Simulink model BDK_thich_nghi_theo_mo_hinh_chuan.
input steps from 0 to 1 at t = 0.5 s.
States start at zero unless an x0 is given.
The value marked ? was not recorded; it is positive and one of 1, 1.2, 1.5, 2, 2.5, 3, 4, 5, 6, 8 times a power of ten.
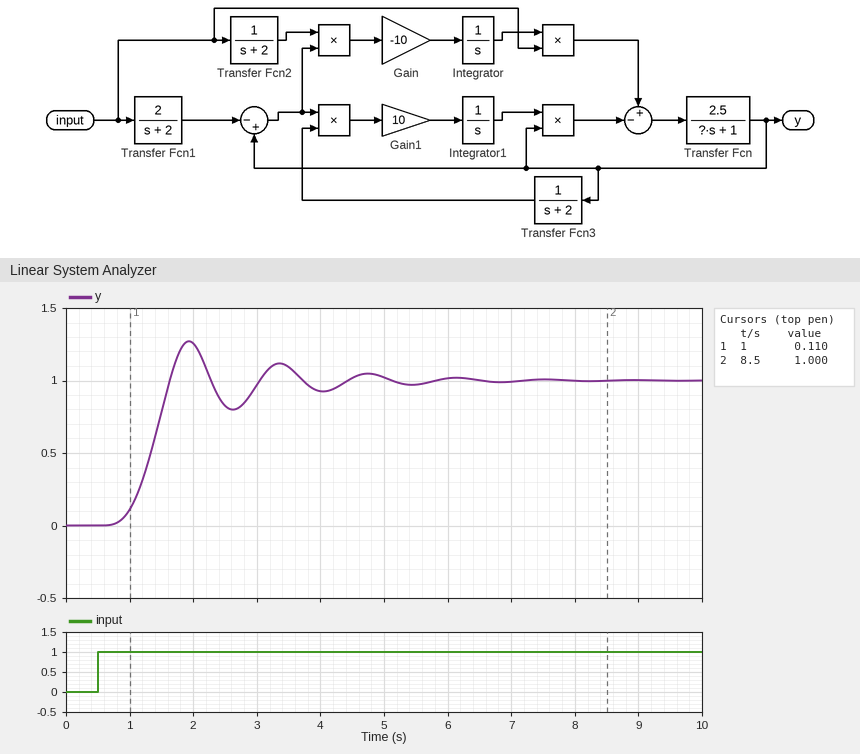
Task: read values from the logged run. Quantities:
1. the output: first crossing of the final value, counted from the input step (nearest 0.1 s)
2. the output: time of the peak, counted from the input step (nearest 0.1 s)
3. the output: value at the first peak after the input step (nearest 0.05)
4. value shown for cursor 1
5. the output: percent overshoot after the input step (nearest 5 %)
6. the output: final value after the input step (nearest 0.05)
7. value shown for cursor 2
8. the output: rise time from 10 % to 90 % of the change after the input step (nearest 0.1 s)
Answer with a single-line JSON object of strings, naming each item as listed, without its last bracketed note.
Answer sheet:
{"the output: first crossing of the final value, counted from the input step": "1.1 s", "the output: time of the peak, counted from the input step": "1.4 s", "the output: value at the first peak after the input step": "1.25", "value shown for cursor 1": "0.110", "the output: percent overshoot after the input step": "25 %", "the output: final value after the input step": "1.00", "value shown for cursor 2": "1.000", "the output: rise time from 10 % to 90 % of the change after the input step": "0.6 s"}
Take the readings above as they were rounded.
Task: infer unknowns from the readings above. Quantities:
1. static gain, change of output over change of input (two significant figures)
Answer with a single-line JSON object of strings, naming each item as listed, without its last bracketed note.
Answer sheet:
{"static gain, change of output over change of input": "1.0"}
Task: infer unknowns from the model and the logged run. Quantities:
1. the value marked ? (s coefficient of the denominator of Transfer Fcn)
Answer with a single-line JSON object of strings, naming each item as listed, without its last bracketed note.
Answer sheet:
{"the value marked ?": "1.2"}
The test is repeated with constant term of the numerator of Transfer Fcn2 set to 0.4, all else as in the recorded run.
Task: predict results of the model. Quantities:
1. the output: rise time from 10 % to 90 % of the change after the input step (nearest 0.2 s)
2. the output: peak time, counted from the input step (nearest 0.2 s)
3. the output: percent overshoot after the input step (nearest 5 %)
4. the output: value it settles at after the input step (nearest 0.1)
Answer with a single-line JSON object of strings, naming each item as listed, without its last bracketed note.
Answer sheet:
{"the output: rise time from 10 % to 90 % of the change after the input step": "0.8 s", "the output: peak time, counted from the input step": "1.8 s", "the output: percent overshoot after the input step": "30 %", "the output: value it settles at after the input step": "1.0"}
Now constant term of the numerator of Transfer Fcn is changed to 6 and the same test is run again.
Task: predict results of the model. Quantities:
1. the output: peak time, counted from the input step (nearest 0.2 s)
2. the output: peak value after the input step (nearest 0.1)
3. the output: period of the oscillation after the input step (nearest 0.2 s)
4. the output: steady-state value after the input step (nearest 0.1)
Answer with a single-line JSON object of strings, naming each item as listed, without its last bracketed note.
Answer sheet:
{"the output: peak time, counted from the input step": "1.0 s", "the output: peak value after the input step": "1.2", "the output: period of the oscillation after the input step": "1.0 s", "the output: steady-state value after the input step": "1.0"}
